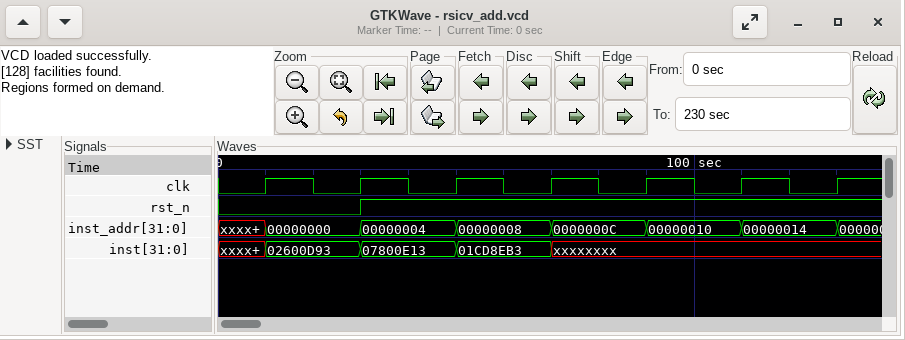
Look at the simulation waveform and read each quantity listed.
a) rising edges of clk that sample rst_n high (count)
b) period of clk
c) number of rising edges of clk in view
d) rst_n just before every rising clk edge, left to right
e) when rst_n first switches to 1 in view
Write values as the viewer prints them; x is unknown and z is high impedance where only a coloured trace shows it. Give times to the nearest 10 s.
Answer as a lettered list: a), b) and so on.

a) 5
b) 20 s
c) 7
d) 0 0 1 1 1 1 1
e) 30 s
